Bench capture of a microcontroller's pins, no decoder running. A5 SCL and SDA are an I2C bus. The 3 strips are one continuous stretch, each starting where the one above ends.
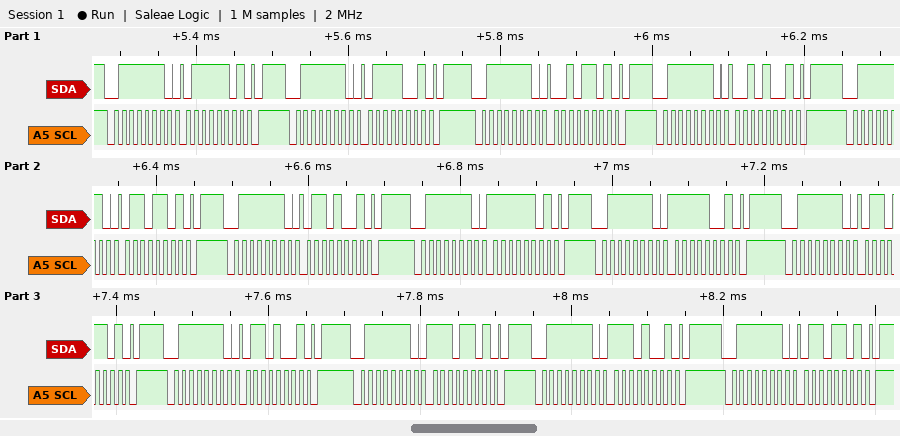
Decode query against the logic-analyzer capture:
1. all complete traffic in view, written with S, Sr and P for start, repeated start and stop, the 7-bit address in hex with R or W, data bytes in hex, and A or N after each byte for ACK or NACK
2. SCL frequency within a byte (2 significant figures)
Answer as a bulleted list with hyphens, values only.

- S 3FW A 7D A P S 3FW A 79 A P S 3FW A 2D A P S 3FW A 29 A P S 3FW A 6D A P S 3FW A 69 A P S 3FW A FD A P S 3FW A F9 A P S 3FW A 6D A P S 3FW A 69 A P S 3FW A ED A P S 3FW A E9 A P S 3FW A 6D A P
- 100 kHz
